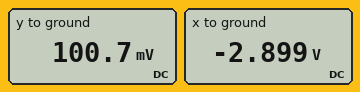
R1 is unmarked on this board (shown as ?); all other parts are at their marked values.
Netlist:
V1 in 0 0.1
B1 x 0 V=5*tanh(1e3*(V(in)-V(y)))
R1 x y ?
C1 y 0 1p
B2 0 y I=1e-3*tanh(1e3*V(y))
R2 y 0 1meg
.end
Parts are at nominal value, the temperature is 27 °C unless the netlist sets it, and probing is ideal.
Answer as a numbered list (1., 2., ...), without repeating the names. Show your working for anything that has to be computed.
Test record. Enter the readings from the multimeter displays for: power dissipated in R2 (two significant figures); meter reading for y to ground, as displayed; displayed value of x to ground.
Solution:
1. (100.7 mV)^2 / 1 MΩ = 10 nW
2. 100.7 mV
3. -2.899 V
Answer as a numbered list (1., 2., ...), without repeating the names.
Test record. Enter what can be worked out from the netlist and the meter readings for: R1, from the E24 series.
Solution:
1. 3 kΩ
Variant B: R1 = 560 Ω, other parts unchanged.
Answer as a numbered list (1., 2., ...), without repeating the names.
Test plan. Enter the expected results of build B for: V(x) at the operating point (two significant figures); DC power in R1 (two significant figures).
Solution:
1. -460 mV
2. 560 µW
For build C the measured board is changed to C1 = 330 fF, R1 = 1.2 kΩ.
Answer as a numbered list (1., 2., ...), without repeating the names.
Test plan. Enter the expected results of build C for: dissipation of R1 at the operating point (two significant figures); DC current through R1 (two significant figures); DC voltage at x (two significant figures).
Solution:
1. 1.2 mW
2. 1.0 mA
3. -1.1 V
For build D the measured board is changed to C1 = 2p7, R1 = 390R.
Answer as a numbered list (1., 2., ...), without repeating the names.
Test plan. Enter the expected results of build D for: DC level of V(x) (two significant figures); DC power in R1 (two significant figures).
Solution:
1. -290 mV
2. 390 µW
